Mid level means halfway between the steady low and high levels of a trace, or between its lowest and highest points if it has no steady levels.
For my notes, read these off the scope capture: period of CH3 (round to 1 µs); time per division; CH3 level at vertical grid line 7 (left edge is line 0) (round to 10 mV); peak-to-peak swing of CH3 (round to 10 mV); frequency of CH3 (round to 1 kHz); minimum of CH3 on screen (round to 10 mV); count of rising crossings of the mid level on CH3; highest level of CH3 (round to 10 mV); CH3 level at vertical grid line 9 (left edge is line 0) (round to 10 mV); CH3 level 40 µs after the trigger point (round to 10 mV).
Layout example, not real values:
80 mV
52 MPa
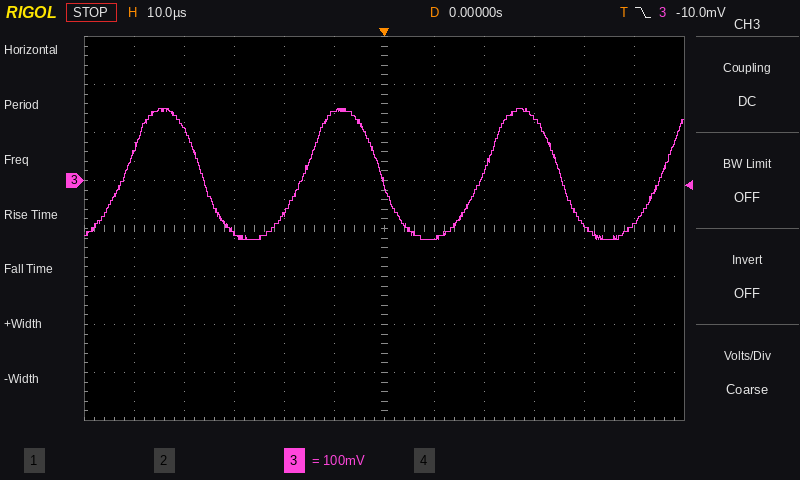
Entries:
36 µs
10 µs
-120 mV
270 mV
28 kHz
-120 mV
4
150 mV
130 mV
-90 mV
